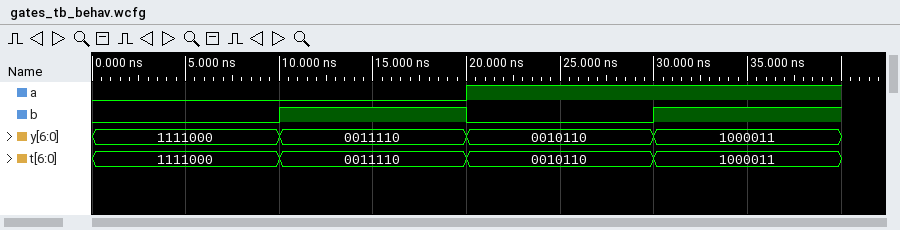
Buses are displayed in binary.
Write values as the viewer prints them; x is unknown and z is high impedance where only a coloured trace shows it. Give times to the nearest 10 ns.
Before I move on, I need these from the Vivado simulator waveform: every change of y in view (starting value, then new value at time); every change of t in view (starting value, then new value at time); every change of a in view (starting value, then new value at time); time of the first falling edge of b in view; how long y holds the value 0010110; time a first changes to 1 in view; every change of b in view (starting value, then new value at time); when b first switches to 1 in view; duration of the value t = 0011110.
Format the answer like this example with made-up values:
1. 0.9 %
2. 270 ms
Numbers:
1. 1111000, 0011110 at 10 ns, 0010110 at 20 ns, 1000011 at 30 ns
2. 1111000, 0011110 at 10 ns, 0010110 at 20 ns, 1000011 at 30 ns
3. 0, 1 at 20 ns
4. 20 ns
5. 10 ns
6. 20 ns
7. 0, 1 at 10 ns, 0 at 20 ns, 1 at 30 ns
8. 10 ns
9. 10 ns
